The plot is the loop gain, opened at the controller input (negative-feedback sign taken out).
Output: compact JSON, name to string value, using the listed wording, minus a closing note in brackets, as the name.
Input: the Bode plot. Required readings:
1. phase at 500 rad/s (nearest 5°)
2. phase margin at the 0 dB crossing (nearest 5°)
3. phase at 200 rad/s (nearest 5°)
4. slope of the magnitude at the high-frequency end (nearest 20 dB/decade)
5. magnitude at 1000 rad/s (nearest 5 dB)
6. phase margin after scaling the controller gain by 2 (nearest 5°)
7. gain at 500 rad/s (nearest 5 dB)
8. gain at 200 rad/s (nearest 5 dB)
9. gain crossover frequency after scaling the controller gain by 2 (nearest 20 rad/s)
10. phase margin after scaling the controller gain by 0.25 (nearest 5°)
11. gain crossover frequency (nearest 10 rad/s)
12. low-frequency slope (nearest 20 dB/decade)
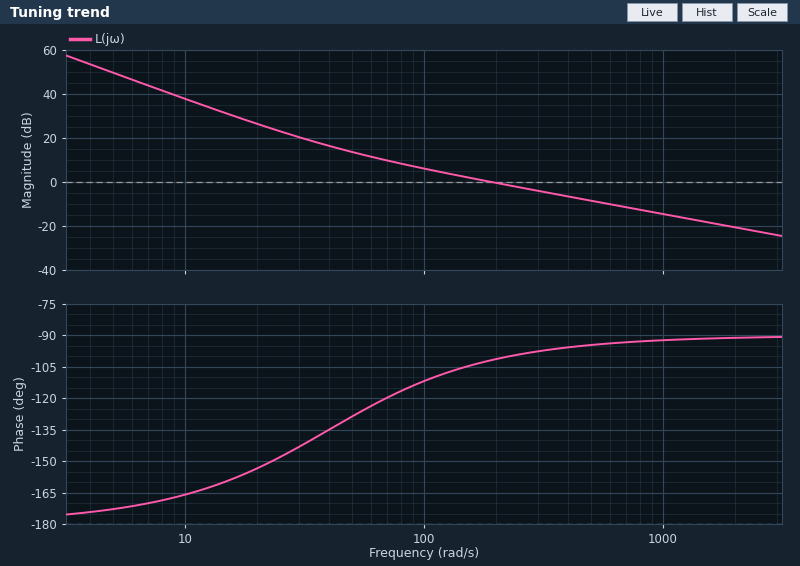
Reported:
{"phase at 500 rad/s": "-95°", "phase margin at the 0 dB crossing": "80°", "phase at 200 rad/s": "-100°", "slope of the magnitude at the high-frequency end": "-20 dB/decade", "magnitude at 1000 rad/s": "-15 dB", "phase margin after scaling the controller gain by 2": "85°", "gain at 500 rad/s": "-10 dB", "gain at 200 rad/s": "0 dB", "gain crossover frequency after scaling the controller gain by 2": "380 rad/s", "phase margin after scaling the controller gain by 0.25": "55°", "gain crossover frequency": "190 rad/s", "low-frequency slope": "-40 dB/decade"}
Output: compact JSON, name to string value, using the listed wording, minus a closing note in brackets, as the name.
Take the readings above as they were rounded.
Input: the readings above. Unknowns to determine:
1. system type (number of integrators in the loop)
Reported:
{"system type": "2"}
